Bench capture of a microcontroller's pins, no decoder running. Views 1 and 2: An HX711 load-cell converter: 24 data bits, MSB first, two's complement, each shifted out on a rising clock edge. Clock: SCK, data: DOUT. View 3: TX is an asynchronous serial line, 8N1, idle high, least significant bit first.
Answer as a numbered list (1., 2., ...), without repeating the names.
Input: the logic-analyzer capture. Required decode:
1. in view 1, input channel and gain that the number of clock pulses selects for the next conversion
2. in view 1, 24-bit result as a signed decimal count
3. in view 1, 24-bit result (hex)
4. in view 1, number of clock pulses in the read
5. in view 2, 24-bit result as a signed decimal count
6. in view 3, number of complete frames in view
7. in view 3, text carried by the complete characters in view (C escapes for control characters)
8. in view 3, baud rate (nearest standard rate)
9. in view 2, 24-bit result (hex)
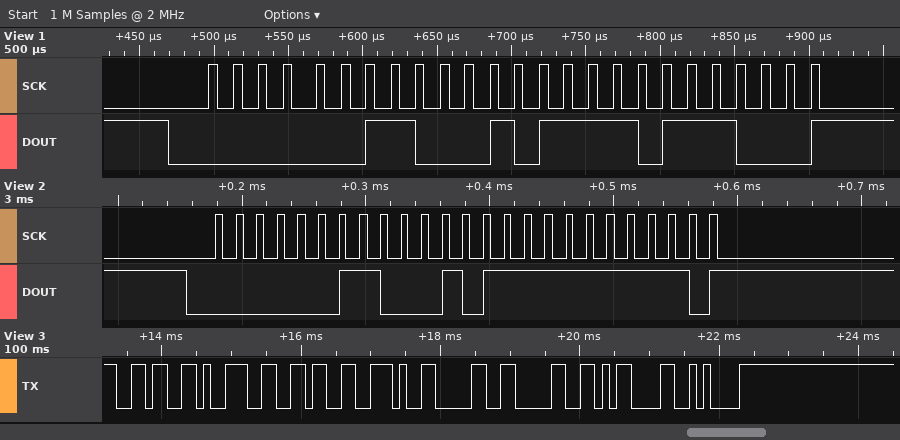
1. channel A, gain 128
2. 202680
3. 0x0317B8
4. 25
5. 202750
6. 8
7. "696.00\r\n"
8. 9600 baud
9. 0x0317FE
